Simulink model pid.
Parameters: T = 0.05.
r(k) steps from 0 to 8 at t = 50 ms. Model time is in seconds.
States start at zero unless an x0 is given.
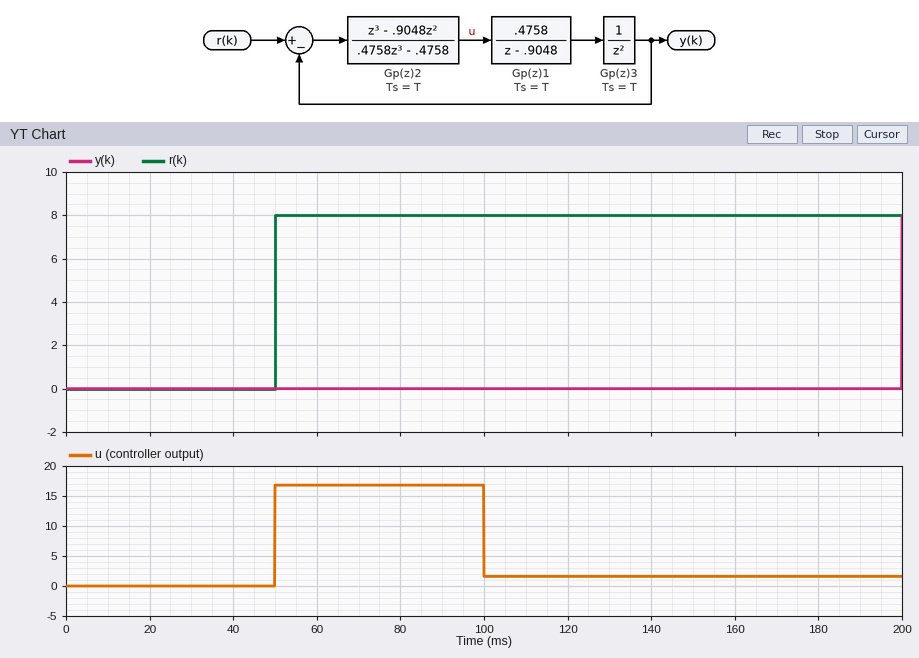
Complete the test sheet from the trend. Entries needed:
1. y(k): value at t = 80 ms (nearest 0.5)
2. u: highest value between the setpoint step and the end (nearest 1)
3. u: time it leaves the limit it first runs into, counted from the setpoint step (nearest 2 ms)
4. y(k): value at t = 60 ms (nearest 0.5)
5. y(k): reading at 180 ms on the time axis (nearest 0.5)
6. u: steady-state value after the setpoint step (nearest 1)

0.0
17
50 ms
0.0
0.0
2
